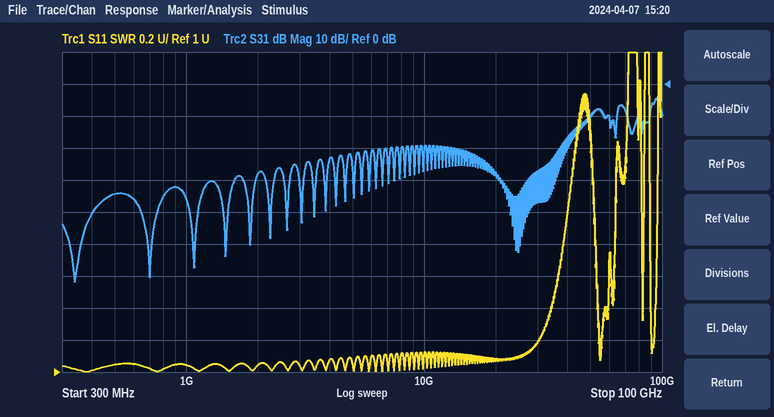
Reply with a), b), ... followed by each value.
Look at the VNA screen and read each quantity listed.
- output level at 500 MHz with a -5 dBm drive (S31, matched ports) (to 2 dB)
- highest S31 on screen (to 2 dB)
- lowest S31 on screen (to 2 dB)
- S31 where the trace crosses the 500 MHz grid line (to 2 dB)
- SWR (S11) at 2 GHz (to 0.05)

a) -40 dBm
b) -4 dB
c) -62 dB
d) -34 dB
e) 1.05
